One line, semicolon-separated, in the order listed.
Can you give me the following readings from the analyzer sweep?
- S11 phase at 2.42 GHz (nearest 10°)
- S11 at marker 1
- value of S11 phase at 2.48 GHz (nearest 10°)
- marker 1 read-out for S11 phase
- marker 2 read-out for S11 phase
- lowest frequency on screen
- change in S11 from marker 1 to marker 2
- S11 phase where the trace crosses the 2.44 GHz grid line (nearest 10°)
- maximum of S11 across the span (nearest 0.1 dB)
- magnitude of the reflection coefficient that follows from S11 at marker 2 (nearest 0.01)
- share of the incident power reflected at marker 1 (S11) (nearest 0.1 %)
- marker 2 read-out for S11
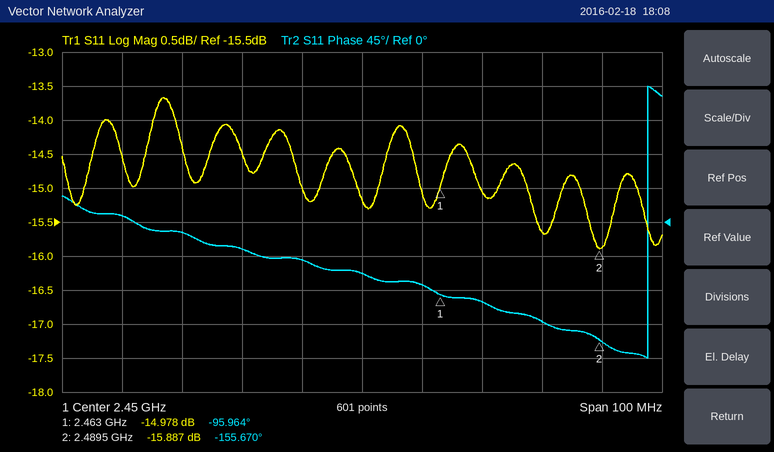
-10°; -14.978 dB; -130°; -95.964°; -155.670°; 2.4 GHz; -0.909 dB; -50°; -13.7 dB; 0.16; 3.2 %; -15.887 dB
